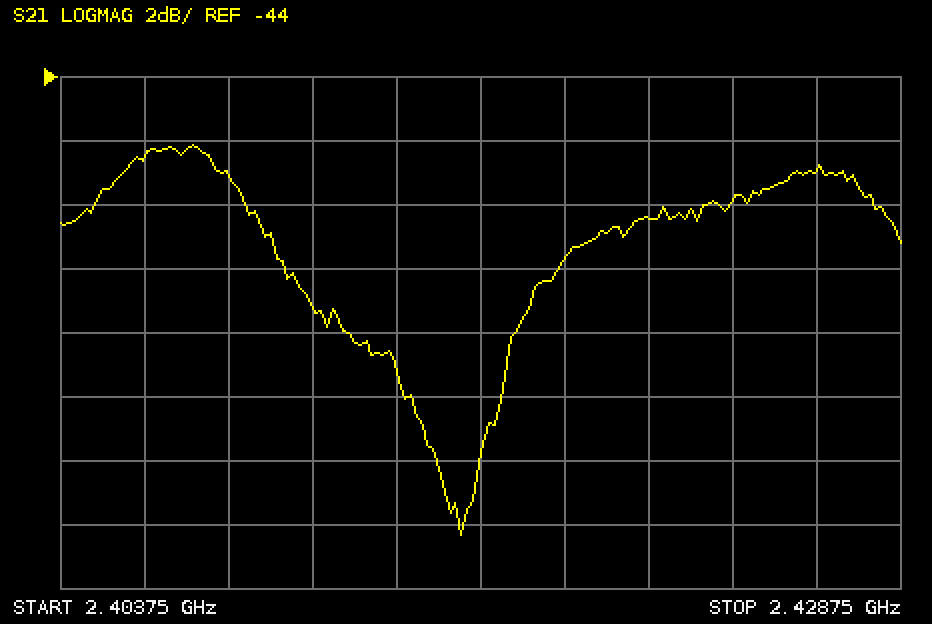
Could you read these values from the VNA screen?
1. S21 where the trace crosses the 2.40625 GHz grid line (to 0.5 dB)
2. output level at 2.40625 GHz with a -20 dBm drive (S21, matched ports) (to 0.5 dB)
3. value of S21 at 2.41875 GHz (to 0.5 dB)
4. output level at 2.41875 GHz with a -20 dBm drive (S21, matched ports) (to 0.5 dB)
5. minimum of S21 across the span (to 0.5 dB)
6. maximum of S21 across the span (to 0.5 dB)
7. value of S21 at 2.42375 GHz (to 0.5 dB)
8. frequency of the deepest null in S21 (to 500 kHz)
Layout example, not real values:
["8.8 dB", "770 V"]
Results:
["-46.5 dB", "-66.5 dBm", "-49.5 dB", "-69.5 dBm", "-58.5 dB", "-46.0 dB", "-48.0 dB", "2.4155 GHz"]
